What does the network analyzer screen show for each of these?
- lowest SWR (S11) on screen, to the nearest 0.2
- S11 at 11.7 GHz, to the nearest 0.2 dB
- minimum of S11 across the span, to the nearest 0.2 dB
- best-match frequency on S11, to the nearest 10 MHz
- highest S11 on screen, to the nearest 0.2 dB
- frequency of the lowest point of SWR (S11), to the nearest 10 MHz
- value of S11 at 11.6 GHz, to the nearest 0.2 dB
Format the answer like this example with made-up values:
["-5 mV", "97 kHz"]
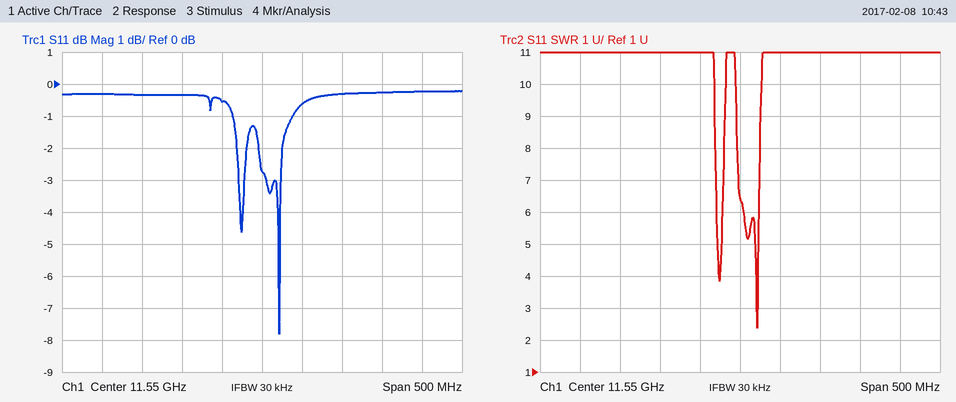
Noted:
["2.4", "-0.2 dB", "-7.8 dB", "11.57 GHz", "-0.2 dB", "11.57 GHz", "-0.6 dB"]
